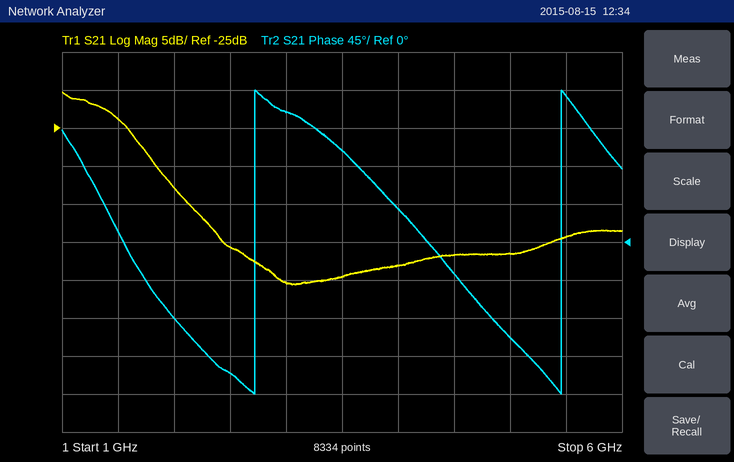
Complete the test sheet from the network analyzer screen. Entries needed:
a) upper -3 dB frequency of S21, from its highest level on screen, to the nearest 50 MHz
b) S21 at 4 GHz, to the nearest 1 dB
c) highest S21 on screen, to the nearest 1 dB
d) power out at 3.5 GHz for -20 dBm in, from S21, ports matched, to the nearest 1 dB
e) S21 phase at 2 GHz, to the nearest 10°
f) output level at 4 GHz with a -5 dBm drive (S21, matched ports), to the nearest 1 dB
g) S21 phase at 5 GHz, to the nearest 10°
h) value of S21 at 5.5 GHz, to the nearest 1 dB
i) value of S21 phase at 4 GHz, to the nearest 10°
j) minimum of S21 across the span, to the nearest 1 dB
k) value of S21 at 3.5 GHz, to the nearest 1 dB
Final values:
1.45 GHz
-43 dB
-20 dB
-65 dBm
-90°
-48 dBm
-110°
-39 dB
40°
-46 dB
-45 dB
